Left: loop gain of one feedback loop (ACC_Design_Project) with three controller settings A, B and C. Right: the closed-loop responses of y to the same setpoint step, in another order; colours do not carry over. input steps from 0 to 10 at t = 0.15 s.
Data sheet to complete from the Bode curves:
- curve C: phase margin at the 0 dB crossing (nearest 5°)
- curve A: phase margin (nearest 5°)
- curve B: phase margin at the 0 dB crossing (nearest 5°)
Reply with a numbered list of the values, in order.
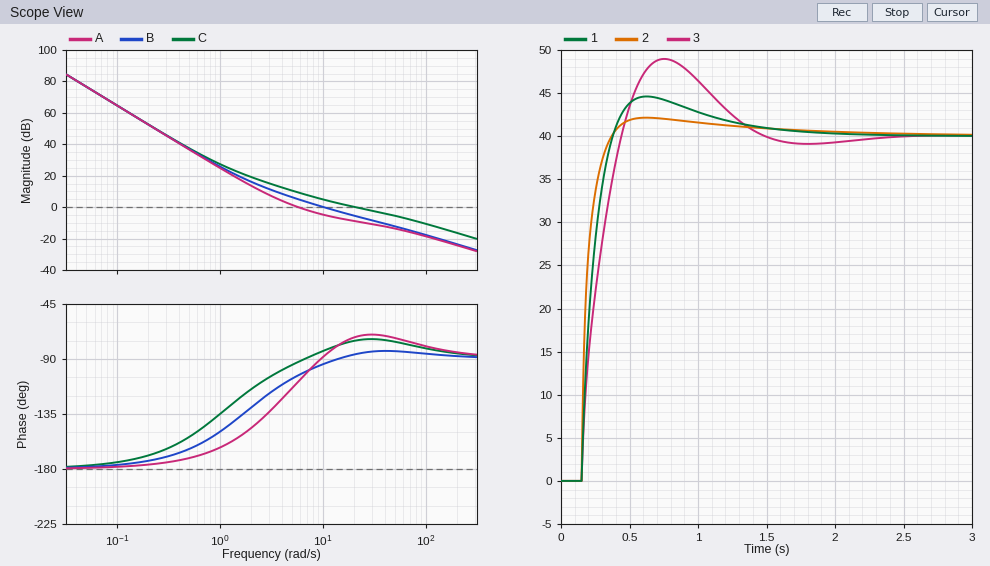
1. 105°
2. 70°
3. 85°
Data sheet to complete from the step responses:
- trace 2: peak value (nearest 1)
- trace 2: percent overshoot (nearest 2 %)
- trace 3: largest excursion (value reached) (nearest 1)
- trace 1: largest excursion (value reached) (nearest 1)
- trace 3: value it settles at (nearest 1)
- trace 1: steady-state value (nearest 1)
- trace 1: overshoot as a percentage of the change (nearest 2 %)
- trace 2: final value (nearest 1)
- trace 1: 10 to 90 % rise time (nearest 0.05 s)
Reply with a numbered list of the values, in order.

1. 42
2. 6 %
3. 49
4. 45
5. 40
6. 40
7. 12 %
8. 40
9. 0.15 s
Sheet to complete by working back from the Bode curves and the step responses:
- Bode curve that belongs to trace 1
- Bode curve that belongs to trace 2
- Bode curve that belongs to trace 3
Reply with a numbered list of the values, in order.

1. B
2. C
3. A
